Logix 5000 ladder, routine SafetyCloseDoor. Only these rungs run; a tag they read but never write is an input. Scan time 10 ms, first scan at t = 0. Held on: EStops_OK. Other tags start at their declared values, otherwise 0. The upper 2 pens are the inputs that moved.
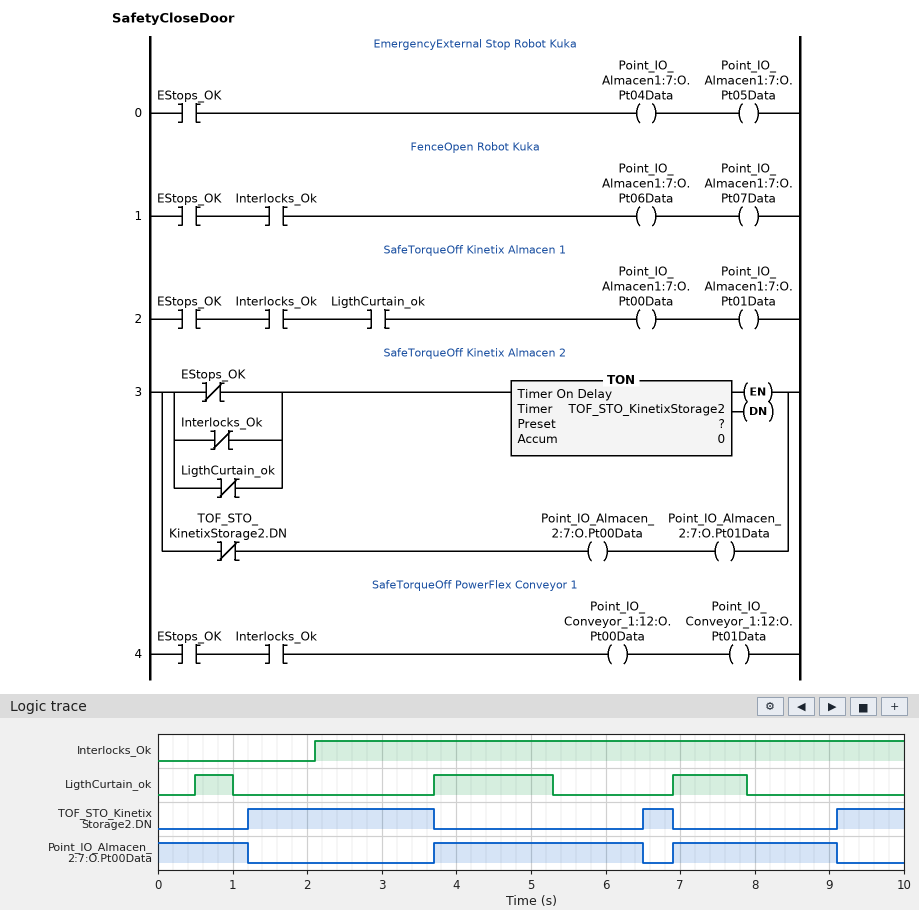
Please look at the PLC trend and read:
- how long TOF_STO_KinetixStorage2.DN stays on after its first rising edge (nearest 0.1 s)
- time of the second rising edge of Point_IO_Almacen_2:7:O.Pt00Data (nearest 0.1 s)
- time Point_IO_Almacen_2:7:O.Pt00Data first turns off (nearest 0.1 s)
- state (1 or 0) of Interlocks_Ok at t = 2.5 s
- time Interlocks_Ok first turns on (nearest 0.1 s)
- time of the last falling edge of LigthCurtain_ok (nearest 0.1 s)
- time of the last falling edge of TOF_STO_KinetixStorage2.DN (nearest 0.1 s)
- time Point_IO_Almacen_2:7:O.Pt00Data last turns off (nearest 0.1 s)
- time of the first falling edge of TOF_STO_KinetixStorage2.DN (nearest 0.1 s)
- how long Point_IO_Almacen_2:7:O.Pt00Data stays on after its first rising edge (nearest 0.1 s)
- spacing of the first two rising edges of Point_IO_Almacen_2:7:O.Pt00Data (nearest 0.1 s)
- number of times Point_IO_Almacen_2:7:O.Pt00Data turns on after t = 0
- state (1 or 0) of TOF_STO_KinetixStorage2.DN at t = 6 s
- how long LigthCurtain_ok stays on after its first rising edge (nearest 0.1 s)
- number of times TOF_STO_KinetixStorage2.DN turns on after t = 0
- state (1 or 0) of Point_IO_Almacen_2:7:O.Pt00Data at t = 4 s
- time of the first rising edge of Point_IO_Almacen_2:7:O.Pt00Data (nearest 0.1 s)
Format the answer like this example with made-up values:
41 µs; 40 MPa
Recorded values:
2.5 s; 6.9 s; 1.2 s; 1; 2.1 s; 7.9 s; 6.9 s; 9.1 s; 3.7 s; 2.8 s; 3.2 s; 2; 0; 0.5 s; 3; 1; 3.7 s
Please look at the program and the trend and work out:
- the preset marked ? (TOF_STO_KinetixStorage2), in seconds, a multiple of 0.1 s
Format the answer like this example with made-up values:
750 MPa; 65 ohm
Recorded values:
1.2 s
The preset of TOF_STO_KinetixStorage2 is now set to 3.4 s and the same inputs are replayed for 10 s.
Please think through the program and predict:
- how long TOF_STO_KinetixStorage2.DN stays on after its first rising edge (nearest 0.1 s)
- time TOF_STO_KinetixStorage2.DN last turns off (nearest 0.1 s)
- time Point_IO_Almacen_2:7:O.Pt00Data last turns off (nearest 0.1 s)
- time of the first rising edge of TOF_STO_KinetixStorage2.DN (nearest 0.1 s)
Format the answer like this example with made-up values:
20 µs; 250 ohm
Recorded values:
0.3 s; 3.7 s; 3.4 s; 3.4 s
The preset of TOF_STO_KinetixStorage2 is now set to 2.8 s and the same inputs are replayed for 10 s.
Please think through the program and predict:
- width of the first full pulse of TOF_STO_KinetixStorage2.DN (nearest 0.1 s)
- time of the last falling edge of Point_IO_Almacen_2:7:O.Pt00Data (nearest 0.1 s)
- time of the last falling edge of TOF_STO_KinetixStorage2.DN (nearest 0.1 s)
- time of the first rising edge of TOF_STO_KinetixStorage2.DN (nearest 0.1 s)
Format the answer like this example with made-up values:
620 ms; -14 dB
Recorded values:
0.9 s; 2.8 s; 3.7 s; 2.8 s
